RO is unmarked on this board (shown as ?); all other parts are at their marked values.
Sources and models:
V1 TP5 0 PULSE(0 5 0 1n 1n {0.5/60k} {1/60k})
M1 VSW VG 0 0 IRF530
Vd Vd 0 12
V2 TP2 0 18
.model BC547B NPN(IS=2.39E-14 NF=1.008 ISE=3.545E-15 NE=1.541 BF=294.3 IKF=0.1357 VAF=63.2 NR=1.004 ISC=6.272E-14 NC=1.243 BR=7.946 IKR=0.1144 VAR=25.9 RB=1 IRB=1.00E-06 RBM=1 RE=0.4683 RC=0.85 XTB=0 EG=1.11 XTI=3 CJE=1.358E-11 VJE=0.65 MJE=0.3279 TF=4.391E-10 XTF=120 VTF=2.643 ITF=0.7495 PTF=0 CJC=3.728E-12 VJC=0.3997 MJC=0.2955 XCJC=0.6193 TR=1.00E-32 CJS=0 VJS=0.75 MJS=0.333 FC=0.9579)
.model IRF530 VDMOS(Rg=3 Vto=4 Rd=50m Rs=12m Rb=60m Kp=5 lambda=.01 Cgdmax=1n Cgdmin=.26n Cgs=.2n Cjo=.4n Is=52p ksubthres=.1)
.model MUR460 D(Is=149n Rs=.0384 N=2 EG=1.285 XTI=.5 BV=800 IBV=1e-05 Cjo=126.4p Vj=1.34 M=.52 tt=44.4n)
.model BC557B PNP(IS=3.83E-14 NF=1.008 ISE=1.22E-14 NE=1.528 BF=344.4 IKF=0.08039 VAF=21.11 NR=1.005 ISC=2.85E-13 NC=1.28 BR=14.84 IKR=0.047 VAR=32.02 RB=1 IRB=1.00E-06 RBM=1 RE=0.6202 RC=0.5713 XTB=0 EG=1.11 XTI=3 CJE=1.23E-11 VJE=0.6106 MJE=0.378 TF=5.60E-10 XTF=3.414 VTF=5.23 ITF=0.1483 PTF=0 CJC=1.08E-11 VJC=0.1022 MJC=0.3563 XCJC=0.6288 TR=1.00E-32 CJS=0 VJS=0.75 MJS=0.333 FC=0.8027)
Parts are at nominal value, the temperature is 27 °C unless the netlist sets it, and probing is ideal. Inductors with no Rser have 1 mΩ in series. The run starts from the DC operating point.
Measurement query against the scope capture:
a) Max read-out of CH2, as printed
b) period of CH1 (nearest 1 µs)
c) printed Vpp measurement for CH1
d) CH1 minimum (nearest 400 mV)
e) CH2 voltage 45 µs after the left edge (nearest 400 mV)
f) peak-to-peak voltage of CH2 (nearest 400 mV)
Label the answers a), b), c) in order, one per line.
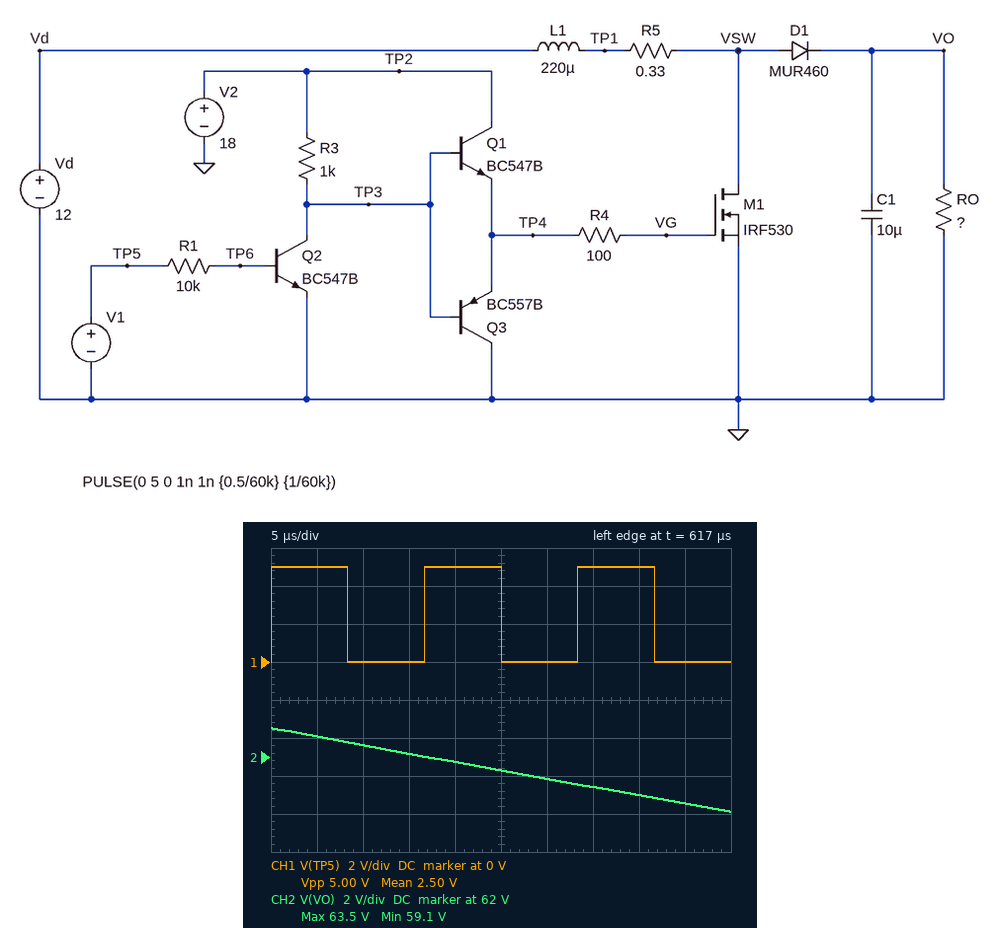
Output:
a) 63.5 V
b) 17 µs
c) 5.00 V
d) 0 V
e) 59.6 V
f) 4.4 V
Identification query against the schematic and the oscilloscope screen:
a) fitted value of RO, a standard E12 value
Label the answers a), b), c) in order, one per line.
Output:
a) 68 Ω
